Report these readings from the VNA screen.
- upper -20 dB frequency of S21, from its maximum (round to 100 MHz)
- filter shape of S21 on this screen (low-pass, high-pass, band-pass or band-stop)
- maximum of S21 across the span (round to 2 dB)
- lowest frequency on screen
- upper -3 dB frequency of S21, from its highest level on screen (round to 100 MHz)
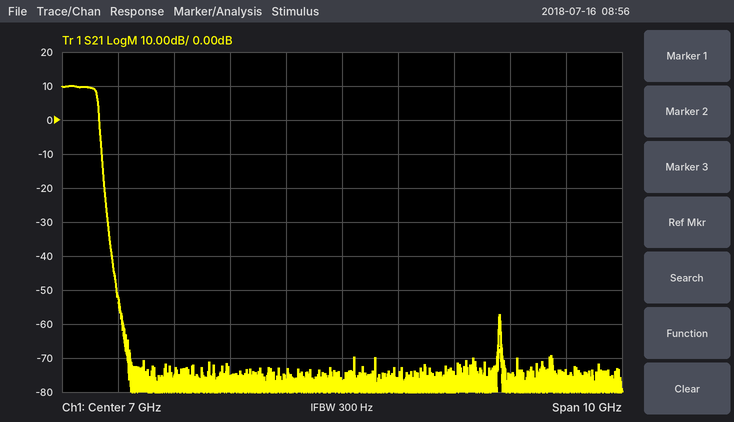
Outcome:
2.7 GHz
low-pass
10 dB
2 GHz
2.6 GHz
